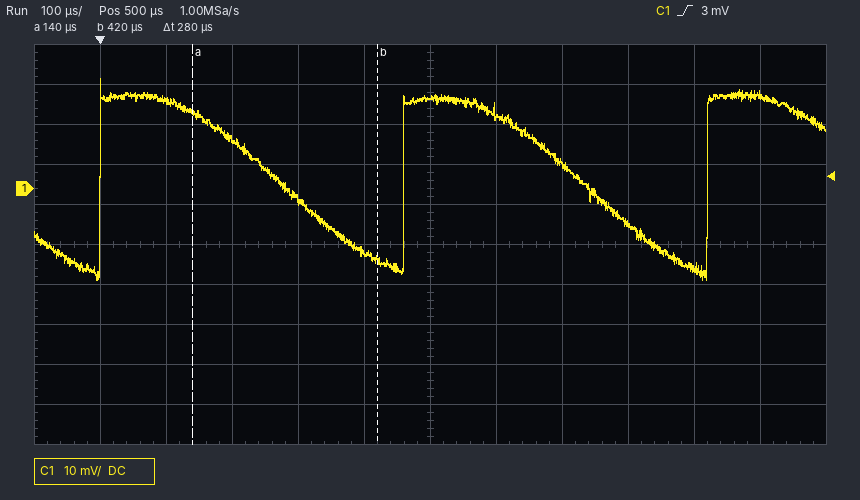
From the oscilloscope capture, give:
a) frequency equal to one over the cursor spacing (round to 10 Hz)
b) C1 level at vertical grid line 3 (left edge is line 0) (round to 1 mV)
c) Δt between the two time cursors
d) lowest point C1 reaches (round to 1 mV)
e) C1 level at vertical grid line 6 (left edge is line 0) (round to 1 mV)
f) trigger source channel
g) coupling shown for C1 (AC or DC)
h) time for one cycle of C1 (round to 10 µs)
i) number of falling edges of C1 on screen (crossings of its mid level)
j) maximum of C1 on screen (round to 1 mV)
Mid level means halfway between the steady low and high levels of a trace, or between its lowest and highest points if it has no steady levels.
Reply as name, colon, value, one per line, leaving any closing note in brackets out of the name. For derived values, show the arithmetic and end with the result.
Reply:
frequency equal to one over the cursor spacing: 1 / 280 µs ≈ 3.57 kHz
C1 level at vertical grid line 3 (left edge is line 0): 12 mV
Δt between the two time cursors: 280 µs
lowest point C1 reaches: -23 mV
C1 level at vertical grid line 6 (left edge is line 0): 23 mV
trigger source channel: C1
coupling shown for C1: DC
time for one cycle of C1: 460 µs
number of falling edges of C1 on screen: 2
maximum of C1 on screen: 28 mV
